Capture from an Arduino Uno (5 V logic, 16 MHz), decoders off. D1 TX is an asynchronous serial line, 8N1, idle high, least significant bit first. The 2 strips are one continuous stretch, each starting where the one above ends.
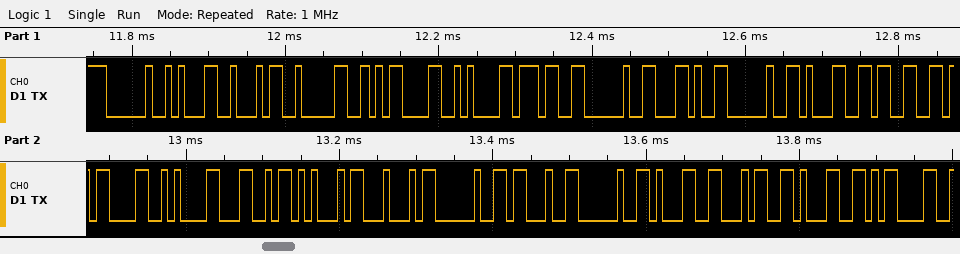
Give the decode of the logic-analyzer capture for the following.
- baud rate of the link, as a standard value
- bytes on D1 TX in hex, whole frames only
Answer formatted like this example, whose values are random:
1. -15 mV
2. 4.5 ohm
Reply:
1. 115200 baud
2. 0x20 0x31 0x34 0x30 0x0D 0x0A 0x37 0x20 0x2C 0x20 0x31 0x33 0x0D 0x0A 0x4C 0x45 0x44 0x20 0x23 0x20 0x31 0x34 0x31 0x0D
